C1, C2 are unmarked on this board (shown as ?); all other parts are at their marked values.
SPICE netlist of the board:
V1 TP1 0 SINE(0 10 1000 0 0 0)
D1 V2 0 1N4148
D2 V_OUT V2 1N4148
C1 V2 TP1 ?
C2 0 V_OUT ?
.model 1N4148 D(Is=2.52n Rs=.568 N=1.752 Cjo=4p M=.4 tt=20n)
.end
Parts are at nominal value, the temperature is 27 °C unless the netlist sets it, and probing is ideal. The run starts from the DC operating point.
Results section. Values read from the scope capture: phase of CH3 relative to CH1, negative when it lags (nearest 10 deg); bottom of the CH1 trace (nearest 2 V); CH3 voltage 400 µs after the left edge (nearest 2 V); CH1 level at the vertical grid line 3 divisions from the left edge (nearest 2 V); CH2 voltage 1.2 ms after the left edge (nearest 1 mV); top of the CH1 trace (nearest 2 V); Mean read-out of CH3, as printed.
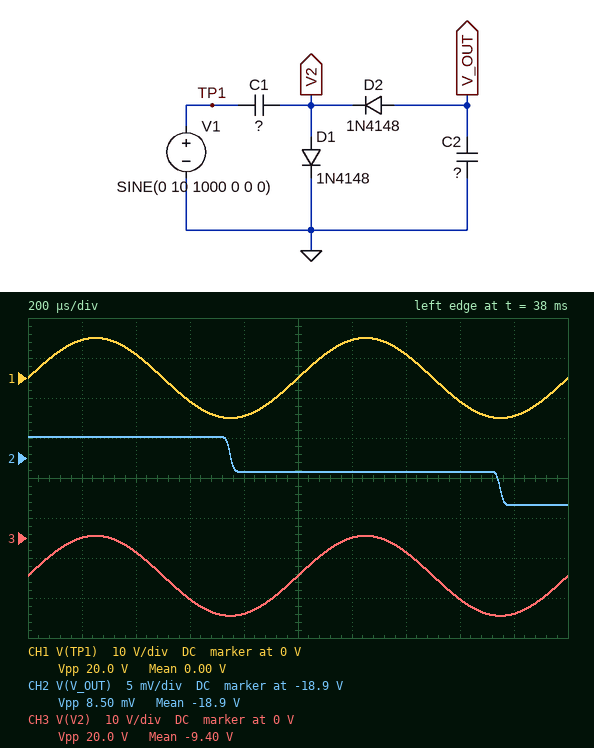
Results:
0 deg
-10 V
-4 V
-6 V
-18.902 V
10 V
-9.40 V
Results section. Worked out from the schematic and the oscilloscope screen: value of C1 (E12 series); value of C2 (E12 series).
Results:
820 nF
2.7 µF
